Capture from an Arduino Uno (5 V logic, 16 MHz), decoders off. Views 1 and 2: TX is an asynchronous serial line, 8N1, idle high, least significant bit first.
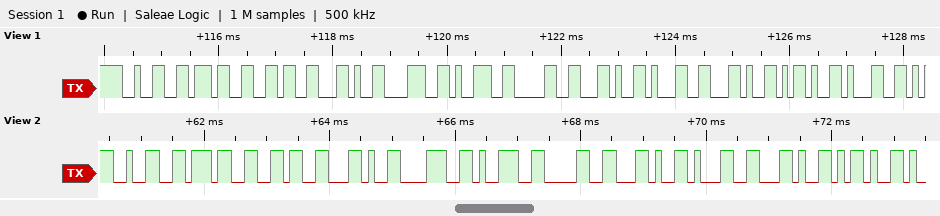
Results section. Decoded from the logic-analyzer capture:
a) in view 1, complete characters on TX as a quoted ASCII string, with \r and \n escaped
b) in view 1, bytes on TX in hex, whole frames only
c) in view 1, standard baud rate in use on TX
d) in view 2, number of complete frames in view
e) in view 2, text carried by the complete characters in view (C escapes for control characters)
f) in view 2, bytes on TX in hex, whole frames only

"276,890,1,-1"
32 37 36 2C 38 39 30 2C 31 2C 2D 31
9600 baud
11
"276,890,1,-"
32 37 36 2C 38 39 30 2C 31 2C 2D
